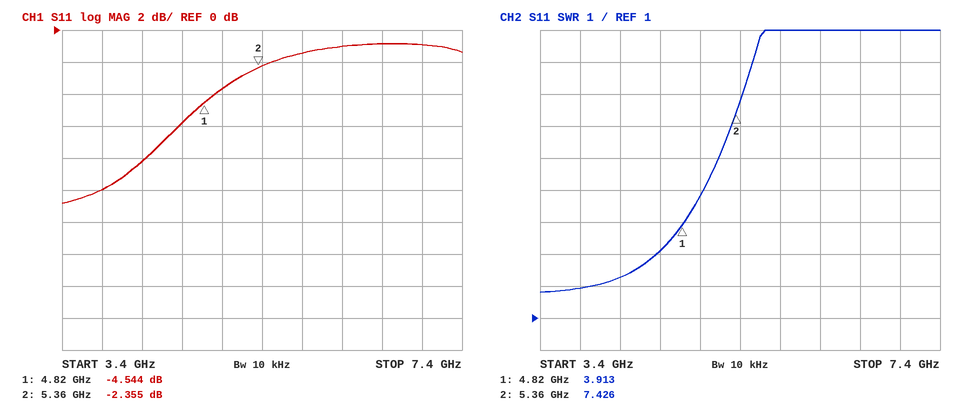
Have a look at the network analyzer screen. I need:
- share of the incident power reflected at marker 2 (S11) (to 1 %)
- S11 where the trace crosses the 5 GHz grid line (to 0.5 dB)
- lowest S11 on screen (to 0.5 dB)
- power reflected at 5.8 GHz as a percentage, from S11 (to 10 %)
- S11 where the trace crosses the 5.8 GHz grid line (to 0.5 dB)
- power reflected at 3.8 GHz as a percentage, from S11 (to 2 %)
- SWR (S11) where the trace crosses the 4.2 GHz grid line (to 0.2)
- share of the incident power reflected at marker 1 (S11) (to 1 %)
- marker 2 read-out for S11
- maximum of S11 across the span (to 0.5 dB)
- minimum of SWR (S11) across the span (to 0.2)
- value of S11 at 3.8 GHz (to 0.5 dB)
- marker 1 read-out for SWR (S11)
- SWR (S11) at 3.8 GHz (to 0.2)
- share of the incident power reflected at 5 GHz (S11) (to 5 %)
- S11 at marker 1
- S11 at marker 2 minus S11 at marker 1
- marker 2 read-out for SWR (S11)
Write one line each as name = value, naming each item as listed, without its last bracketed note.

share of the incident power reflected at marker 2 (S11) = 58 %
S11 where the trace crosses the 5 GHz grid line = -3.5 dB
lowest S11 on screen = -11.0 dB
power reflected at 5.8 GHz as a percentage, from S11 = 70 %
S11 where the trace crosses the 5.8 GHz grid line = -1.5 dB
power reflected at 3.8 GHz as a percentage, from S11 = 10 %
SWR (S11) where the trace crosses the 4.2 GHz grid line = 2.2
share of the incident power reflected at marker 1 (S11) = 35 %
marker 2 read-out for S11 = -2.355 dB
maximum of S11 across the span = -1.0 dB
minimum of SWR (S11) across the span = 1.8
value of S11 at 3.8 GHz = -10.0 dB
marker 1 read-out for SWR = 3.913
SWR (S11) at 3.8 GHz = 2.0
share of the incident power reflected at 5 GHz (S11) = 45 %
S11 at marker 1 = -4.544 dB
S11 at marker 2 minus S11 at marker 1 = 2.189 dB
marker 2 read-out for SWR = 7.426
